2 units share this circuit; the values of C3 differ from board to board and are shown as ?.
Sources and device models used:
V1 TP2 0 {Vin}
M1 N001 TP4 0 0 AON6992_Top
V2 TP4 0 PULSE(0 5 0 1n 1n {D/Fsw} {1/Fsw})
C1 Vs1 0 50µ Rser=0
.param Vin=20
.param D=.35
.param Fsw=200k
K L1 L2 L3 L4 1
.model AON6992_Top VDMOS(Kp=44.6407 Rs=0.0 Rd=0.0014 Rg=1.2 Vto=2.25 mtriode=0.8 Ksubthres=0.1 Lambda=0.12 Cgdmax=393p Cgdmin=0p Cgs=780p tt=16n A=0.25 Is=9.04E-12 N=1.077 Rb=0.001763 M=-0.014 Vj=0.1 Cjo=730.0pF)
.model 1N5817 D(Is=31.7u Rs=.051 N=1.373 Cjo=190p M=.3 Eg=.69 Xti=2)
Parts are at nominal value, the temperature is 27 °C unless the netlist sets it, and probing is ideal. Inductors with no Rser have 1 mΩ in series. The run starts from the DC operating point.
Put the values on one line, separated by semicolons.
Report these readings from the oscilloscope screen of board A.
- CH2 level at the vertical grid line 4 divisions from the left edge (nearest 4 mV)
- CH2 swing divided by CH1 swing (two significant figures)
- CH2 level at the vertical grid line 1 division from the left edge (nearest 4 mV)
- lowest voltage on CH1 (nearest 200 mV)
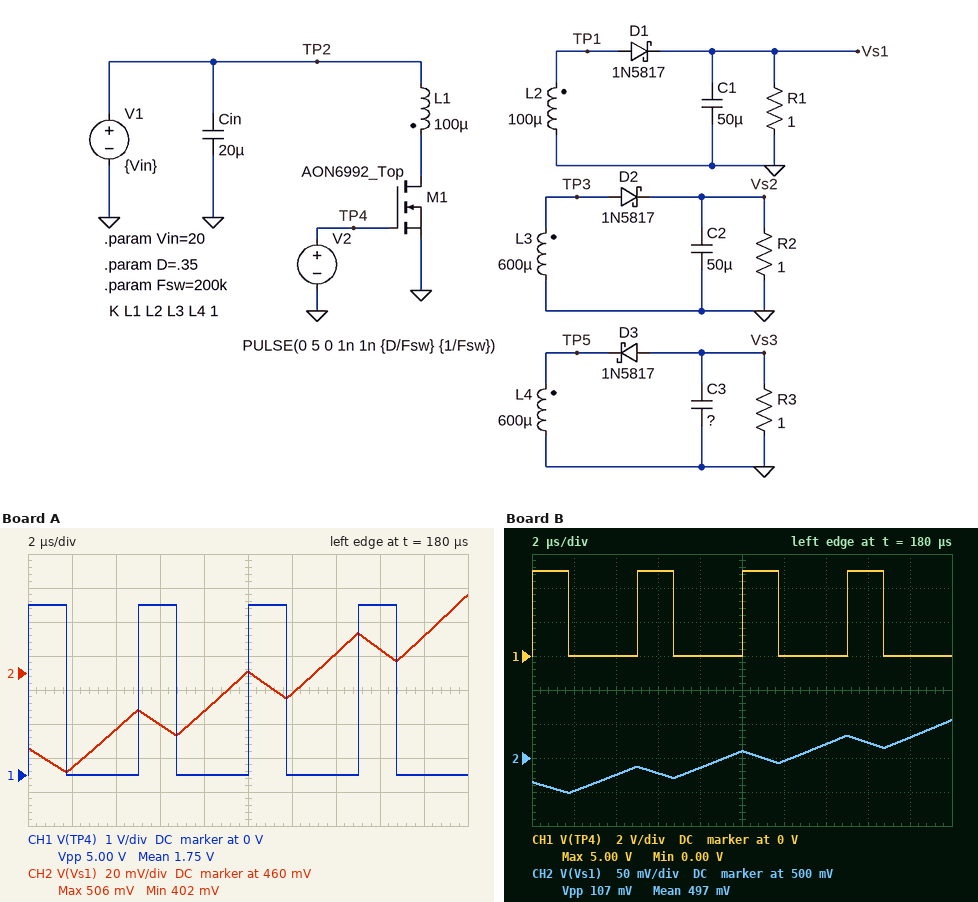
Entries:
436 mV; 0.021; 404 mV; 0 V
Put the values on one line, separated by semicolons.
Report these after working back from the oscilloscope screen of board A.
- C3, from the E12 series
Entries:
56 µF
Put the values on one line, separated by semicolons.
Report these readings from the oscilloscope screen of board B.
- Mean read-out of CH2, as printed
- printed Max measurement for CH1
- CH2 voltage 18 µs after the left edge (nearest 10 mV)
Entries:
497 mV; 5.00 V; 530 mV
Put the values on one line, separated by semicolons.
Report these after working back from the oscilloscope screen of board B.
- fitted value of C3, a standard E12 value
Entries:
27 µF
